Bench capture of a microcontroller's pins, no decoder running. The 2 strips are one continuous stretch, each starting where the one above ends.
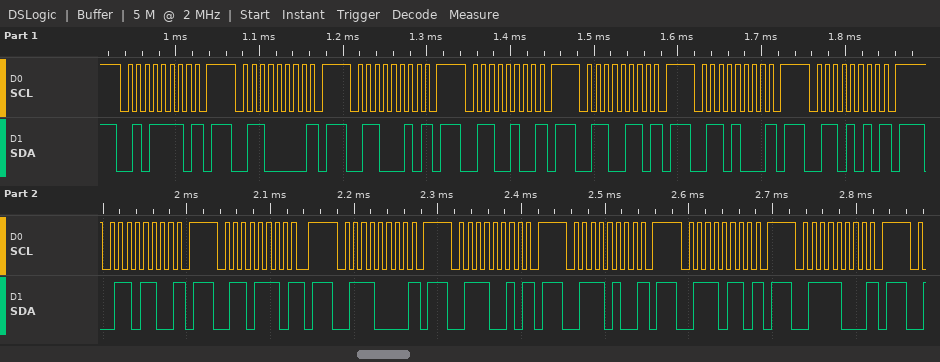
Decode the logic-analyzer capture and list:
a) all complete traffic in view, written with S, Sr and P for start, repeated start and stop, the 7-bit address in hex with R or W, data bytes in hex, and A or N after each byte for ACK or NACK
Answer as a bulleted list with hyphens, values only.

- S 2FW N P S 30W N P S 31W N P S 32W N P S 33W N P S 34W N P S 35W N P S 36W N P S 37W N P S 38W N P S 39W N P S 3AW N P S 3BW N P S 3CW N P
